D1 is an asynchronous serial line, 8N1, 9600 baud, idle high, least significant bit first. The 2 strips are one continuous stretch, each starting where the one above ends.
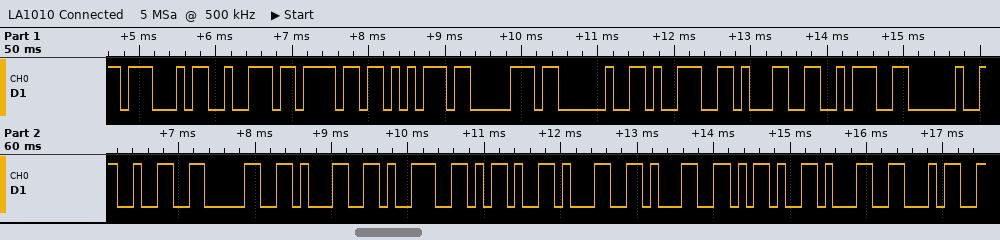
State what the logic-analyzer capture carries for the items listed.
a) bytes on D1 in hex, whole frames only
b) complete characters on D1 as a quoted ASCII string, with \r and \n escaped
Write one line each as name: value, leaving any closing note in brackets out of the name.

bytes on D1 in hex, whole frames only: 47 72 6F 75 70 20 39 31 3A 20 32 30 31 39 2D 31 31 2D 31 34
complete characters on D1 as a quoted ASCII string, with \r and \n escaped: "Group 91: 2019-11-14"
